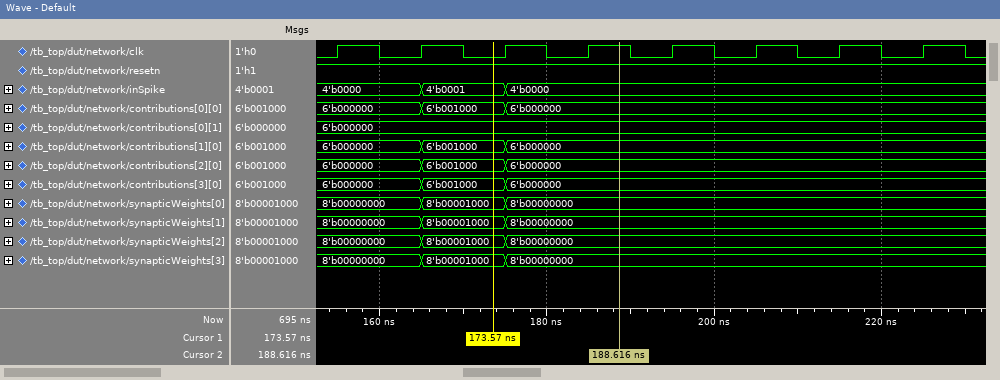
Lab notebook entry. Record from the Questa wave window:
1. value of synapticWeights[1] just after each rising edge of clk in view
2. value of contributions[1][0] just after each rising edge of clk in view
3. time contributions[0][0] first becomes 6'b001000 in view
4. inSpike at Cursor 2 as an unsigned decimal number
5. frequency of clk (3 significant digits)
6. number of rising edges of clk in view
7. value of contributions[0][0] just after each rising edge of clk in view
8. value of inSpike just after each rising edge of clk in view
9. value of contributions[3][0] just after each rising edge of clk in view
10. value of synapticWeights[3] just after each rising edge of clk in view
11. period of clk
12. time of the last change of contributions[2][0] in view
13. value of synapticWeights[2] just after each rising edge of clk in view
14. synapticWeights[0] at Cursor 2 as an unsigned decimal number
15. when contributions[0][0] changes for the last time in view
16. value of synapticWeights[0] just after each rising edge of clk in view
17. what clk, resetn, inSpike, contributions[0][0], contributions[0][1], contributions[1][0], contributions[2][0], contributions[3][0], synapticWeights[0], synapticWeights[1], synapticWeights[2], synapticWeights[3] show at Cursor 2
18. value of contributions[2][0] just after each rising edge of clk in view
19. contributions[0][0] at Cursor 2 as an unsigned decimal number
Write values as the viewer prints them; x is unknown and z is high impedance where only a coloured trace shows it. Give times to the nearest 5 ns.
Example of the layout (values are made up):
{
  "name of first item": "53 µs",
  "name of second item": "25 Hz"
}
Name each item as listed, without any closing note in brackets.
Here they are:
{
  "value of synapticWeights[1] just after each rising edge of clk in view": "8'b00000000, 8'b00001000, 8'b00000000, 8'b00000000, 8'b00000000, 8'b00000000, 8'b00000000, 8'b00000000",
  "value of contributions[1][0] just after each rising edge of clk in view": "6'b000000, 6'b001000, 6'b000000, 6'b000000, 6'b000000, 6'b000000, 6'b000000, 6'b000000",
  "time contributions[0][0] first becomes 6'b001000 in view": "165 ns",
  "inSpike at Cursor 2 as an unsigned decimal number": "0",
  "frequency of clk": "100 MHz",
  "number of rising edges of clk in view": "8",
  "value of contributions[0][0] just after each rising edge of clk in view": "6'b000000, 6'b001000, 6'b000000, 6'b000000, 6'b000000, 6'b000000, 6'b000000, 6'b000000",
  "value of inSpike just after each rising edge of clk in view": "4'b0000, 4'b0001, 4'b0000, 4'b0000, 4'b0000, 4'b0000, 4'b0000, 4'b0000",
  "value of contributions[3][0] just after each rising edge of clk in view": "6'b000000, 6'b001000, 6'b000000, 6'b000000, 6'b000000, 6'b000000, 6'b000000, 6'b000000",
  "value of synapticWeights[3] just after each rising edge of clk in view": "8'b00000000, 8'b00001000, 8'b00000000, 8'b00000000, 8'b00000000, 8'b00000000, 8'b00000000, 8'b00000000",
  "period of clk": "10 ns",
  "time of the last change of contributions[2][0] in view": "175 ns",
  "value of synapticWeights[2] just after each rising edge of clk in view": "8'b00000000, 8'b00001000, 8'b00000000, 8'b00000000, 8'b00000000, 8'b00000000, 8'b00000000, 8'b00000000",
  "synapticWeights[0] at Cursor 2 as an unsigned decimal number": "0",
  "when contributions[0][0] changes for the last time in view": "175 ns",
  "value of synapticWeights[0] just after each rising edge of clk in view": "8'b00000000, 8'b00001000, 8'b00000000, 8'b00000000, 8'b00000000, 8'b00000000, 8'b00000000, 8'b00000000",
  "what clk, resetn, inSpike, contributions[0][0], contributions[0][1], contributions[1][0], contributions[2][0], contributions[3][0], synapticWeights[0], synapticWeights[1], synapticWeights[2], synapticWeights[3] show at Cursor 2": "clk=1, resetn=1, inSpike=4'b0000, contributions[0][0]=6'b000000, contributions[0][1]=6'b000000, contributions[1][0]=6'b000000, contributions[2][0]=6'b000000, contributions[3][0]=6'b000000, synapticWeights[0]=8'b00000000, synapticWeights[1]=8'b00000000, synapticWeights[2]=8'b00000000, synapticWeights[3]=8'b00000000",
  "value of contributions[2][0] just after each rising edge of clk in view": "6'b000000, 6'b001000, 6'b000000, 6'b000000, 6'b000000, 6'b000000, 6'b000000, 6'b000000",
  "contributions[0][0] at Cursor 2 as an unsigned decimal number": "0"
}
